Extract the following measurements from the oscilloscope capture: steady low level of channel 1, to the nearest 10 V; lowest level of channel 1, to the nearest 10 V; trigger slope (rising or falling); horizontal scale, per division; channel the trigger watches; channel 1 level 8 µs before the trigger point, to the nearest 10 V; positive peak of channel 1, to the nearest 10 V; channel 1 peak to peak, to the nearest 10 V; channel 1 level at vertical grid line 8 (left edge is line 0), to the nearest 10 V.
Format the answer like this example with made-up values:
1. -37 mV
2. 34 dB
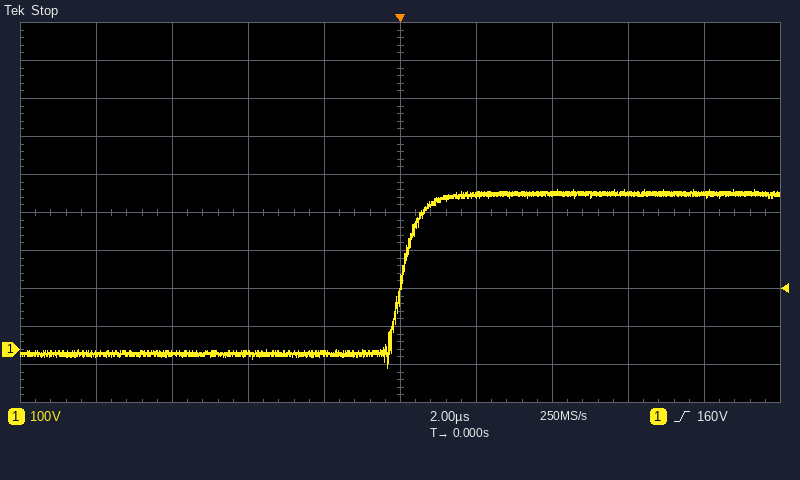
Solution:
1. -10 V
2. -50 V
3. rising
4. 2 µs
5. channel 1
6. -10 V
7. 420 V
8. 470 V
9. 410 V
